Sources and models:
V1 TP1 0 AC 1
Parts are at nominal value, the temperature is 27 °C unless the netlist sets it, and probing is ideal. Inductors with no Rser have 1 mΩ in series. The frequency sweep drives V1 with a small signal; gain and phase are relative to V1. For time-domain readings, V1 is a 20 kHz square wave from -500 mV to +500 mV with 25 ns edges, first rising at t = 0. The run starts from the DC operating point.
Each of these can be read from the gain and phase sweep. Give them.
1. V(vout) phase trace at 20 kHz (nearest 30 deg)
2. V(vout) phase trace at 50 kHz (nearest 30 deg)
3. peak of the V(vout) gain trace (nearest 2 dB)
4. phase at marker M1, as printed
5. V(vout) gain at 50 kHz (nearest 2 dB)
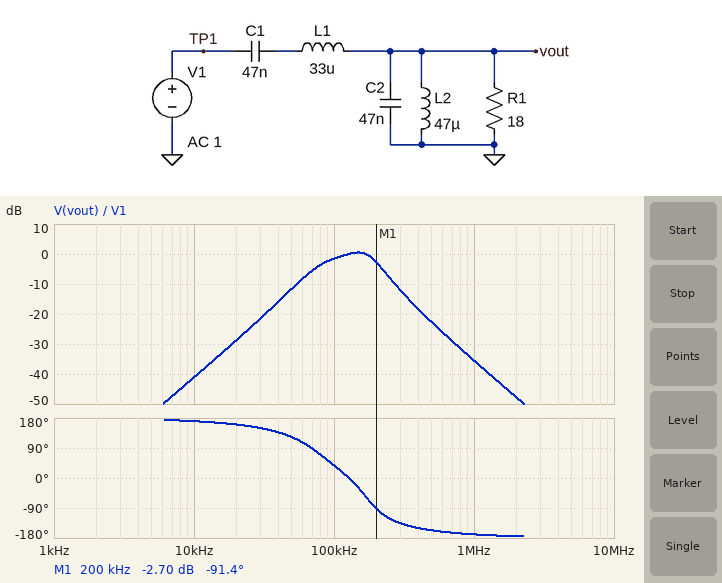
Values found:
150 deg
120 deg
0 dB
-91.4 deg
-12 dB
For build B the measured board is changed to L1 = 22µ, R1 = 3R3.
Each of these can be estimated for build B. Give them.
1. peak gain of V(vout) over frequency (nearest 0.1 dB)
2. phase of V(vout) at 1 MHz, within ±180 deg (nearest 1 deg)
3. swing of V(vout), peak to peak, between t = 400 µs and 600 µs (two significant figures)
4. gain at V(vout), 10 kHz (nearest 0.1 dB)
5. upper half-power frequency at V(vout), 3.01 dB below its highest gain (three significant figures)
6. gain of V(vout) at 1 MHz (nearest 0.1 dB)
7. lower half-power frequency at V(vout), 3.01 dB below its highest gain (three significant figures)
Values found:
0 dB
-133 deg
230 mV
-43.6 dB
170 kHz
-35.0 dB
146 kHz
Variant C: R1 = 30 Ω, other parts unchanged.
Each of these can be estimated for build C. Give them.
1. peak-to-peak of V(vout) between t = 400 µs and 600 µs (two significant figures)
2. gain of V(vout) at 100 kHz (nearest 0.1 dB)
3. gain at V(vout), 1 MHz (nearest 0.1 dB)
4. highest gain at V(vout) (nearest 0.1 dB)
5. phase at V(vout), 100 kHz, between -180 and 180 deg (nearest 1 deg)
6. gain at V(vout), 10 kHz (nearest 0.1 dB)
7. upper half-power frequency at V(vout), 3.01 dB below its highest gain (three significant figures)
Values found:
870 mV
-0.3 dB
-35.4 dB
2.9 dB
25 deg
-41.0 dB
214 kHz
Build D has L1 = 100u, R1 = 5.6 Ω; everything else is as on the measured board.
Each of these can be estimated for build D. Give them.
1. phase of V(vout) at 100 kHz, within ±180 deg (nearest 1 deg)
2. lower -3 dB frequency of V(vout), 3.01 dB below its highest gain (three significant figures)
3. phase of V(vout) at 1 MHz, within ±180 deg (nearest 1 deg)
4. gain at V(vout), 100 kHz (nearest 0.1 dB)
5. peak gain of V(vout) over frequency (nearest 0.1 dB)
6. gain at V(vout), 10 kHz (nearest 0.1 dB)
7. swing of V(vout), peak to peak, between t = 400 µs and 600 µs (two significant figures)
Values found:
-78 deg
68.5 kHz
-148 deg
-14.5 dB
0.1 dB
-42.0 dB
170 mV
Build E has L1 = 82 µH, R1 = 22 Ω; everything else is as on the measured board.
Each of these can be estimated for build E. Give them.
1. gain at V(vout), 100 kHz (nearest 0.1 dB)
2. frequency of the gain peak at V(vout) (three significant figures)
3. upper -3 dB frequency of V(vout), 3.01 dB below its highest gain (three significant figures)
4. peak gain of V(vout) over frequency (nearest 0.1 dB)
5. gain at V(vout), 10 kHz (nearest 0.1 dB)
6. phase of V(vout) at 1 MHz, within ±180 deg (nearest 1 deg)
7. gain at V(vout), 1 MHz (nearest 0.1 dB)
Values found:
-2.6 dB
70.2 kHz
93.1 kHz
1.3 dB
-41.0 dB
-171 deg
-43.5 dB
